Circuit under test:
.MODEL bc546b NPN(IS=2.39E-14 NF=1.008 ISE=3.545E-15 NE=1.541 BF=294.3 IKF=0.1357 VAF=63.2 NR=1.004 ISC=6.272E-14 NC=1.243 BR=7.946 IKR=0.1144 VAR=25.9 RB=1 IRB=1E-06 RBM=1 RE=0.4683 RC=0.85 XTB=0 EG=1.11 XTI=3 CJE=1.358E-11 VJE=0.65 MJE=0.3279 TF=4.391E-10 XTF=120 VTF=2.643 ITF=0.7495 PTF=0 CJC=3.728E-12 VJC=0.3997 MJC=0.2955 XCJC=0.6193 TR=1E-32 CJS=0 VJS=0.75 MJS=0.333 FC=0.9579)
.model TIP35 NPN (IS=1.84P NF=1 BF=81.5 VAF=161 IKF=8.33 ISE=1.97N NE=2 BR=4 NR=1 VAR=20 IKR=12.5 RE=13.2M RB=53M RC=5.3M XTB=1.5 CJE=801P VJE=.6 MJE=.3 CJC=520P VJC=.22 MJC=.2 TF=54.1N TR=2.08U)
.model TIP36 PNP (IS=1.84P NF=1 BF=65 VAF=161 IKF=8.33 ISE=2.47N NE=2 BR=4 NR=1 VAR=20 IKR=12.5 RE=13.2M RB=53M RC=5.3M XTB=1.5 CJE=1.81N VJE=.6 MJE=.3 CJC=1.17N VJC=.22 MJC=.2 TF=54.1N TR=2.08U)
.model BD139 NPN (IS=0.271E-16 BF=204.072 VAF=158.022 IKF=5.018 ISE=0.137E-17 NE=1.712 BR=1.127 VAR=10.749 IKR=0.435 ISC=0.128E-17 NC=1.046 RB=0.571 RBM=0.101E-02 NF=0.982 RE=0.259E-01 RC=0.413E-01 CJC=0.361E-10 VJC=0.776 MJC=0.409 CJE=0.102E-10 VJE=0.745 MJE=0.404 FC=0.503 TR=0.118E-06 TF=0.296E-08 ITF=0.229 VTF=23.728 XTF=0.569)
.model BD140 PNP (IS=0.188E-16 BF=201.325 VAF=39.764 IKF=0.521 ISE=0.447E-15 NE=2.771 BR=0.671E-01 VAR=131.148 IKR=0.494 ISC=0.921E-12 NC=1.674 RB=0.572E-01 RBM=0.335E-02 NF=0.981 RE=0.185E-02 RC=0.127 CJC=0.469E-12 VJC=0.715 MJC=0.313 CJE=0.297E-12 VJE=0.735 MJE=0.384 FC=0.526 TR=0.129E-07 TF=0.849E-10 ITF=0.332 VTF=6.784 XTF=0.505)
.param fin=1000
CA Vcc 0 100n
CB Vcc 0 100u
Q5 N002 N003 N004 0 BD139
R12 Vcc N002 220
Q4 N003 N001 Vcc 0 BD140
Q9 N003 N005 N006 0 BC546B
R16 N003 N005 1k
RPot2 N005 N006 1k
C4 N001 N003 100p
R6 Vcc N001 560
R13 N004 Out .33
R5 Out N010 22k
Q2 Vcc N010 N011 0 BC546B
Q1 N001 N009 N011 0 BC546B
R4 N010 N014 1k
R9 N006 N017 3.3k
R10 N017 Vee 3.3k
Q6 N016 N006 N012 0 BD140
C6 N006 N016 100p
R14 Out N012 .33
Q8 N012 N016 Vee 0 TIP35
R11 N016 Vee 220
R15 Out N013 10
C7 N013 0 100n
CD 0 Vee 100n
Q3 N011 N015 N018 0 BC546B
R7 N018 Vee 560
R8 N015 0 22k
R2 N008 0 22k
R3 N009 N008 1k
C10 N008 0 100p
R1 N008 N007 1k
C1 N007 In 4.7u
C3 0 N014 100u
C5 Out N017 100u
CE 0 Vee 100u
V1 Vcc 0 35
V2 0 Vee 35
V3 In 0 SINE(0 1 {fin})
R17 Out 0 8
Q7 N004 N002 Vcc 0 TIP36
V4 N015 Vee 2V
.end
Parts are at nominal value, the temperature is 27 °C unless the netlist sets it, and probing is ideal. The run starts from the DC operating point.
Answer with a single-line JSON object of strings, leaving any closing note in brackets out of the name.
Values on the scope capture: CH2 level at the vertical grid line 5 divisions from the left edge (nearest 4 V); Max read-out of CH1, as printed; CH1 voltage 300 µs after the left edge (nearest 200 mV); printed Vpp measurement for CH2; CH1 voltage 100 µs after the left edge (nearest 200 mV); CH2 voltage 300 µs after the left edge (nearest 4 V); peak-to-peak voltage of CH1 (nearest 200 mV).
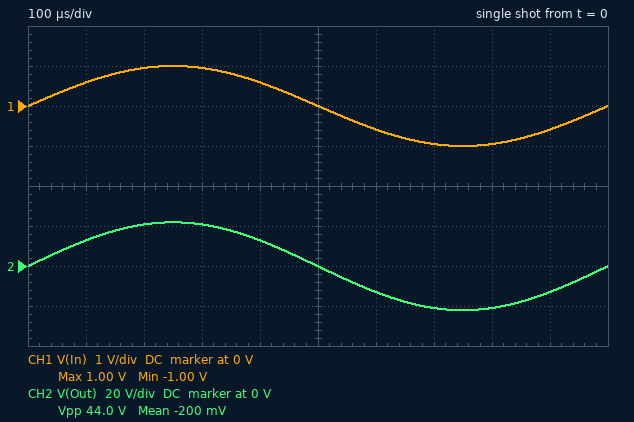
{"CH2 level at the vertical grid line 5 divisions from the left edge": "0 V", "Max read-out of CH1, as printed": "1.00 V", "CH1 voltage 300 µs after the left edge": "1.0 V", "printed Vpp measurement for CH2": "44.0 V", "CH1 voltage 100 µs after the left edge": "600 mV", "CH2 voltage 300 µs after the left edge": "20 V", "peak-to-peak voltage of CH1": "2.0 V"}
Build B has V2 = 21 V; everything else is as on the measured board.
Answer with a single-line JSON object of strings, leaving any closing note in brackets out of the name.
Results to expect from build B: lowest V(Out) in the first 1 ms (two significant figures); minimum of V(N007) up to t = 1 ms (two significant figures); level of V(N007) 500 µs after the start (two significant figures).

{"lowest V(Out) in the first 1 ms": "-19 V", "minimum of V(N007) up to t = 1 ms": "-1.1 V", "level of V(N007) 500 µs after the start": "-76 mV"}
